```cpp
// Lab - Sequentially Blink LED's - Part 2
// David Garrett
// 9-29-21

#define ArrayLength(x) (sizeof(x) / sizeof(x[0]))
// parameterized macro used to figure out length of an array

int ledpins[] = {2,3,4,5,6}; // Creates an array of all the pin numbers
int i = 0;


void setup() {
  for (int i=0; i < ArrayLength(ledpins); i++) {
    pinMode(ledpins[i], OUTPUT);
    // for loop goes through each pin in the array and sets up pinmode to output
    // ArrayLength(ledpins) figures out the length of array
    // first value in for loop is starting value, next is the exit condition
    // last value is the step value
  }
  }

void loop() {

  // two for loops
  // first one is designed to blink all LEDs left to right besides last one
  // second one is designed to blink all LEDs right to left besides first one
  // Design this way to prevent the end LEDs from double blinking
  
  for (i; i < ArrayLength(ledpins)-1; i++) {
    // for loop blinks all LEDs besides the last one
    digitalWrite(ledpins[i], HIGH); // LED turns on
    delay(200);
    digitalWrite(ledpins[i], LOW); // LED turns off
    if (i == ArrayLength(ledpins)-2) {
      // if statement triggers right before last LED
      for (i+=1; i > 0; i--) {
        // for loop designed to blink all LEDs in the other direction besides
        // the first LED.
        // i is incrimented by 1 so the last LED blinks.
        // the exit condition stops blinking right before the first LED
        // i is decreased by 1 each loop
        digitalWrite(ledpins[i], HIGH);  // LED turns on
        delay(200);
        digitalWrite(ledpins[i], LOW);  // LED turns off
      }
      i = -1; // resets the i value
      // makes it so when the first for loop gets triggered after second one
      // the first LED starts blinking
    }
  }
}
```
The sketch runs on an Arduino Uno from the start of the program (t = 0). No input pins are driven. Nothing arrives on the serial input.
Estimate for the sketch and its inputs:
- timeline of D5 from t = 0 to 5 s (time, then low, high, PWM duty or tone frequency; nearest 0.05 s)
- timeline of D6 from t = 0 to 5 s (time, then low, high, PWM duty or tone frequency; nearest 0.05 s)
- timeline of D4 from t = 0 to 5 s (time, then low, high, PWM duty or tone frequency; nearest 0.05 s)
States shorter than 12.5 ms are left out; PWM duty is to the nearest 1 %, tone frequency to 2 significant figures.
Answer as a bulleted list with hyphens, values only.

- 0 s low; 0.6 s high; 0.8 s low; 1 s high; 1.2 s low; 2.2 s high; 2.4 s low; 2.6 s high; 2.8 s low; 3.8 s high; 4 s low; 4.2 s high; 4.4 s low
- 0 s low; 0.8 s high; 1 s low; 2.4 s high; 2.6 s low; 4 s high; 4.2 s low
- 0 s low; 0.4 s high; 0.6 s low; 1.2 s high; 1.4 s low; 2 s high; 2.2 s low; 2.8 s high; 3 s low; 3.6 s high; 3.8 s low; 4.4 s high; 4.6 s low
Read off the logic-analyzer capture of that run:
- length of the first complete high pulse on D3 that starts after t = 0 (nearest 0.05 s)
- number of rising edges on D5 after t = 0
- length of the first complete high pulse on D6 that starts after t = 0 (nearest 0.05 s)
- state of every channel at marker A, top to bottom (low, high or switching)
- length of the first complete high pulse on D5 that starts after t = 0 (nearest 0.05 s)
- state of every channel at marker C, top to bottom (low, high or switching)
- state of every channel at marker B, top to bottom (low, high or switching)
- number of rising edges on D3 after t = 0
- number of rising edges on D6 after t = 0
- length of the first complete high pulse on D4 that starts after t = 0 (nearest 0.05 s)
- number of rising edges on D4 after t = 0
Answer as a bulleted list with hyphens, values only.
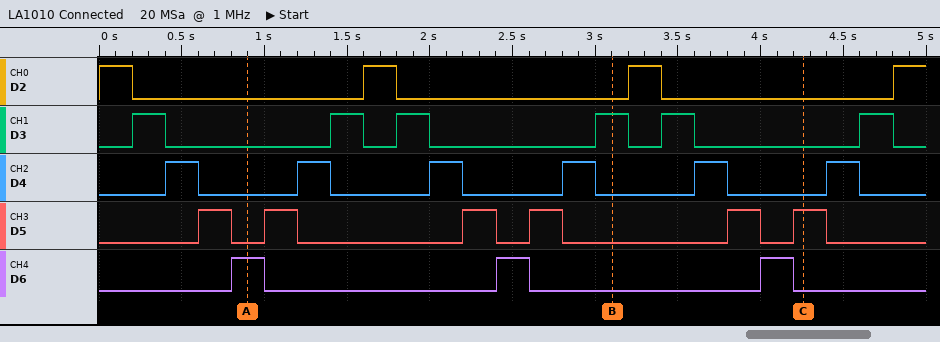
- 0.20 s
- 6
- 0.20 s
- D2 low, D3 low, D4 low, D5 low, D6 high
- 0.20 s
- D2 low, D3 low, D4 low, D5 high, D6 low
- D2 low, D3 high, D4 low, D5 low, D6 low
- 6
- 3
- 0.20 s
- 6
